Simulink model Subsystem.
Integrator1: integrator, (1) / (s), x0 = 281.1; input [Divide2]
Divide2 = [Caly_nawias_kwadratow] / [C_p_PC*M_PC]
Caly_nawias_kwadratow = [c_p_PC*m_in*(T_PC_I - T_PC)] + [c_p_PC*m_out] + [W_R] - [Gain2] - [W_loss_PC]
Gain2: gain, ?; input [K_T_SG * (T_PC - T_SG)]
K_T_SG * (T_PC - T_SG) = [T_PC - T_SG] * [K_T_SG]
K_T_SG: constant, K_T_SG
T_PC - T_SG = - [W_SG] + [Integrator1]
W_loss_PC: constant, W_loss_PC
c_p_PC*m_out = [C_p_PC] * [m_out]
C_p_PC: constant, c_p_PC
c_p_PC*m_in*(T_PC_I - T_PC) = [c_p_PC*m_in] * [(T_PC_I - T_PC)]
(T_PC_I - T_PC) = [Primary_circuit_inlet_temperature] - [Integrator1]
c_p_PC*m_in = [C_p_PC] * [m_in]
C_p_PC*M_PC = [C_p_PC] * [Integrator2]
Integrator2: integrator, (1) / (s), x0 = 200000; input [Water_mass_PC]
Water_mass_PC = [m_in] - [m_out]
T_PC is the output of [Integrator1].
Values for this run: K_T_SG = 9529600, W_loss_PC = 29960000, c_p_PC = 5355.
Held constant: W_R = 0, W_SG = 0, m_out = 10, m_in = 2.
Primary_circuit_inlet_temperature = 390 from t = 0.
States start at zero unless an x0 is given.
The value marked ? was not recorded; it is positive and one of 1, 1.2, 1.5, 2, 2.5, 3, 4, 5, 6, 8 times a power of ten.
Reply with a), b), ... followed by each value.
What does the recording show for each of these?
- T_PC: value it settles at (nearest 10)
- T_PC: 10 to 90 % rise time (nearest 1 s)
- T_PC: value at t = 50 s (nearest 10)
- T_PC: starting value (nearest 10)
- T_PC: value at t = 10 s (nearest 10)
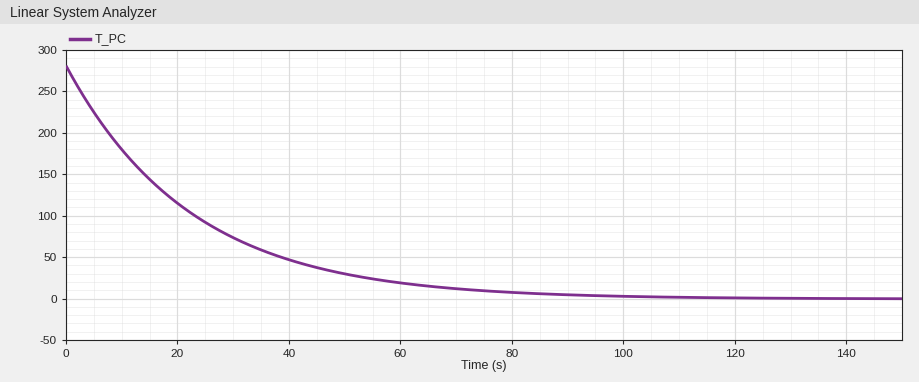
a) 0
b) 49 s
c) 30
d) 280
e) 180
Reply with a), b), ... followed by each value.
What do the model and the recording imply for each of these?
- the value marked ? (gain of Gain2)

a) 5
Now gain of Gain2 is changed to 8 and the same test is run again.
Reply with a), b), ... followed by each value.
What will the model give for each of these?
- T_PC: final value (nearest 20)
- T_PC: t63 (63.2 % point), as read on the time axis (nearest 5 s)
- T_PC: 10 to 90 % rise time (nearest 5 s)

a) 0
b) 15 s
c) 30 s
